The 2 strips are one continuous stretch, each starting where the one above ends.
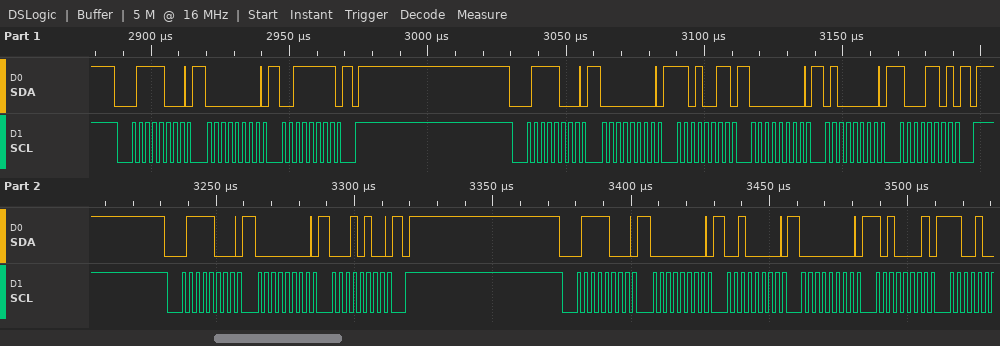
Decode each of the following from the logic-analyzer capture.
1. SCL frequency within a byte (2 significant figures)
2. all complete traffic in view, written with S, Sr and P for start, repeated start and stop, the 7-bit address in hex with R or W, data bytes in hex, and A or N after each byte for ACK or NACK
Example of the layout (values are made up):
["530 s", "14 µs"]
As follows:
["400 kHz", "S 3CW A 00 A 3F A P S 3CW A 00 A D3 A 00 A 40 A 8D A P S 3CW A 00 A 14 A P S 3CW A 00 A 20 A 00 A A1 A"]
